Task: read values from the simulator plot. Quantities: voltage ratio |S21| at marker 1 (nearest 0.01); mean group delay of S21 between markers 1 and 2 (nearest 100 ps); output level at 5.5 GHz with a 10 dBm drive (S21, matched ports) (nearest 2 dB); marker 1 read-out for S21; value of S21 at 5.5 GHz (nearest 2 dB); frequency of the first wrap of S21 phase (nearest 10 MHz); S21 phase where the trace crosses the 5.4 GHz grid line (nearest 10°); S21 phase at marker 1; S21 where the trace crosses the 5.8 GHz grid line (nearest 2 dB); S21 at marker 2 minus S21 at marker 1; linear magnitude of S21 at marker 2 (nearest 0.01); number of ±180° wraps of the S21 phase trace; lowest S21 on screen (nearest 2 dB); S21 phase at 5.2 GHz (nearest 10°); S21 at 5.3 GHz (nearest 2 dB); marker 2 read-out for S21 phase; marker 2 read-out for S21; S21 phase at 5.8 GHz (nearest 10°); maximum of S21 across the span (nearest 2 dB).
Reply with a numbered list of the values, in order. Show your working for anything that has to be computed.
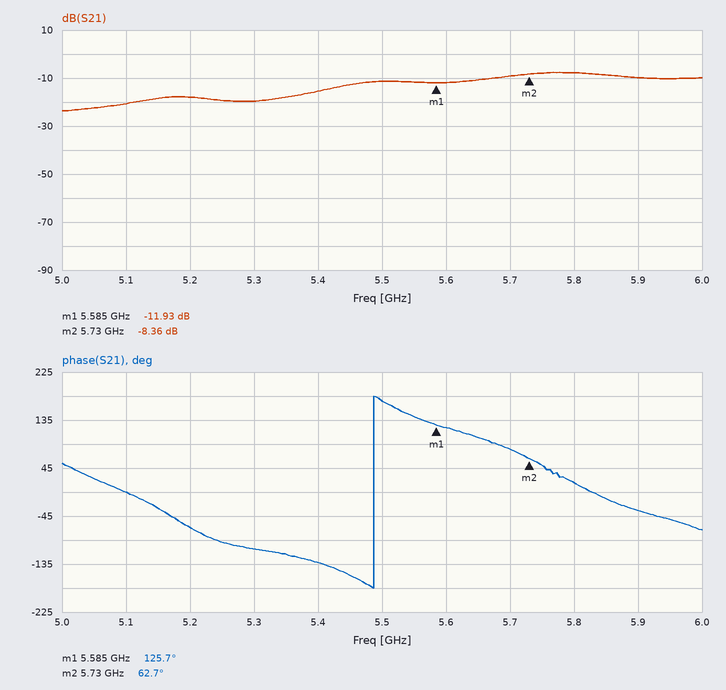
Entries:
1. 10^(-11.93/20) ≈ 0.25
2. −(62.7° − (125.7°))/(360° × 145 MHz) ≈ 1.2 ns
3. 10 dBm + (-12 dB) = -2 dBm
4. -11.93 dB
5. -12 dB
6. 5.49 GHz
7. -130°
8. 125.7°
9. -8 dB
10. -8.36 − (-11.93) = 3.57 dB
11. 10^(-8.36/20) ≈ 0.38
12. 1
13. -24 dB
14. -70°
15. -20 dB
16. 62.7°
17. -8.36 dB
18. 20°
19. -8 dB
